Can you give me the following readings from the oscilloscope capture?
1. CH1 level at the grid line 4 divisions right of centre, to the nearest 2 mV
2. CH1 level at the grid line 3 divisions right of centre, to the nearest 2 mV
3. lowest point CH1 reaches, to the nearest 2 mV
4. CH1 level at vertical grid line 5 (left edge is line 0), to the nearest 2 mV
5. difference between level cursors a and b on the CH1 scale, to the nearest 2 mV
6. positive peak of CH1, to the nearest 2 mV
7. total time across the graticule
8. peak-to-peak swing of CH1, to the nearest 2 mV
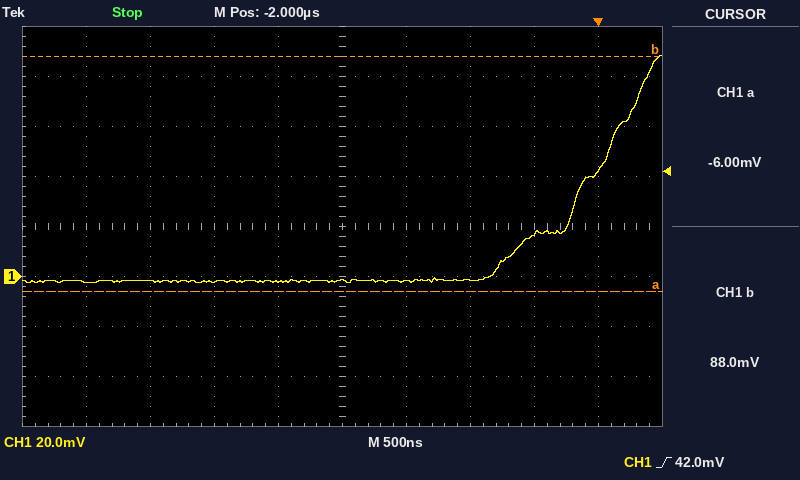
42 mV
18 mV
-2 mV
-2 mV
94 mV
88 mV
5 µs
90 mV
